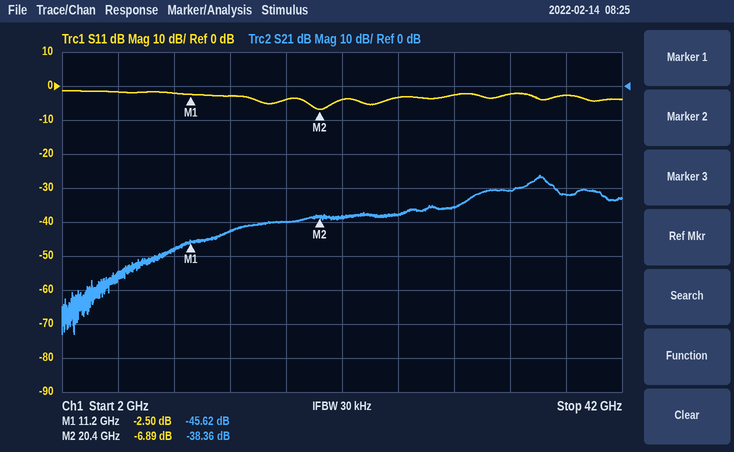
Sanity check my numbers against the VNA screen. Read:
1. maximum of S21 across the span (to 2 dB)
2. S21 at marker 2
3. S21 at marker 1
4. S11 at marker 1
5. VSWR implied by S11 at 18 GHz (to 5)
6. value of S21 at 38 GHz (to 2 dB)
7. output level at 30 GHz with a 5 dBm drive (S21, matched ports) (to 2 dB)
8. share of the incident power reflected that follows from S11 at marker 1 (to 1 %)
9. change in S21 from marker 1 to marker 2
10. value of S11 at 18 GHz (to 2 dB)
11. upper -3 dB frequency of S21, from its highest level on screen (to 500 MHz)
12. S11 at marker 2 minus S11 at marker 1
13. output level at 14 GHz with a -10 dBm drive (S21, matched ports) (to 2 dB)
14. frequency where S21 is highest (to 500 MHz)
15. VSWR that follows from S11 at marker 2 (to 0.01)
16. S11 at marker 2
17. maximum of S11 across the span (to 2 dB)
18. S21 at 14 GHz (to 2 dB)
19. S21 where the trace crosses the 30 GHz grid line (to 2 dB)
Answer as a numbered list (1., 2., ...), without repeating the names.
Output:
1. -26 dB
2. -38.36 dB
3. -45.62 dB
4. -2.50 dB
5. 5
6. -32 dB
7. -30 dBm
8. 56 %
9. 7.26 dB
10. -4 dB
11. 37.0 GHz
12. -4.39 dB
13. -52 dBm
14. 36.0 GHz
15. 2.65
16. -6.89 dB
17. -2 dB
18. -42 dB
19. -36 dB
